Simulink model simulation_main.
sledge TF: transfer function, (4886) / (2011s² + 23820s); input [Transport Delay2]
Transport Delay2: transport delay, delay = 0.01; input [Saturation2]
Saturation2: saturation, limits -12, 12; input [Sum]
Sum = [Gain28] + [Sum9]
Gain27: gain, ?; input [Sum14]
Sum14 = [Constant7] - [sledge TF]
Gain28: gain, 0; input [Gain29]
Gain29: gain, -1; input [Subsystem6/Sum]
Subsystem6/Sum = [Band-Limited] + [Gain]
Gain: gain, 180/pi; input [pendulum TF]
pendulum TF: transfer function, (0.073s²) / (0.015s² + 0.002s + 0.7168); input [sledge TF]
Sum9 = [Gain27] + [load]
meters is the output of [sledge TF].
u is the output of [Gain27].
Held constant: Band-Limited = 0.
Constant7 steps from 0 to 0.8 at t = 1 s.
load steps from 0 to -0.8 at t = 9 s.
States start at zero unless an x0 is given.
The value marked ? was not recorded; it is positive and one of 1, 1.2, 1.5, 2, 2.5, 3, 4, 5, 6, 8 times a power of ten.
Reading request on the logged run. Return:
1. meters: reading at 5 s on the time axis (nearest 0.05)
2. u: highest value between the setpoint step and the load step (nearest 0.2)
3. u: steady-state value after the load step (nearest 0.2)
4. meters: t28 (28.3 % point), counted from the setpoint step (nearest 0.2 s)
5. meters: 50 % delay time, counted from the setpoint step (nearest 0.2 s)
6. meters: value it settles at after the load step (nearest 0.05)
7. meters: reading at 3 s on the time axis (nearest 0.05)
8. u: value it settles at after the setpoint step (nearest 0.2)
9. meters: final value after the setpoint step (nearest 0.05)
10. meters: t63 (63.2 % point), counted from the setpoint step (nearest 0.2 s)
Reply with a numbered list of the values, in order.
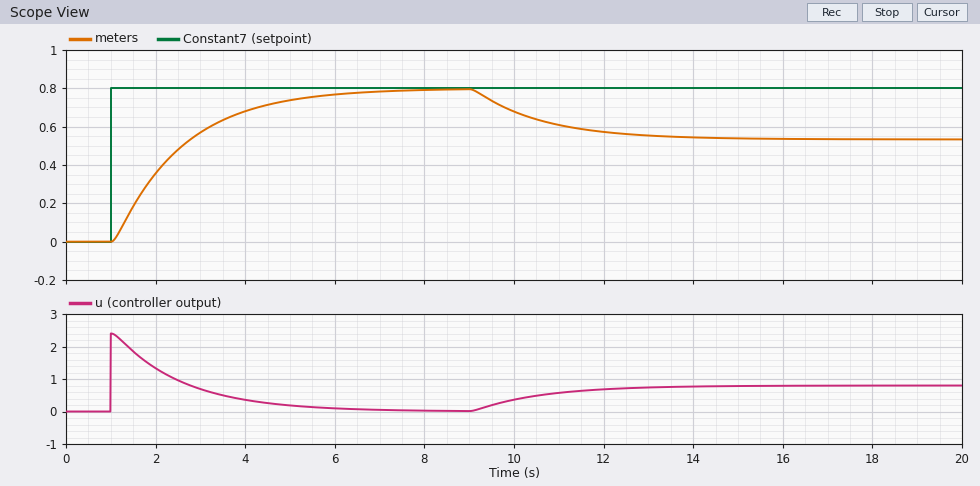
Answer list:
1. 0.75
2. 2.4
3. 0.8
4. 0.6 s
5. 1.2 s
6. 0.55
7. 0.55
8. 0.0
9. 0.80
10. 1.6 s
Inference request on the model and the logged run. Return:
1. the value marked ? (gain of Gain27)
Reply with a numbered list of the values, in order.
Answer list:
1. 3
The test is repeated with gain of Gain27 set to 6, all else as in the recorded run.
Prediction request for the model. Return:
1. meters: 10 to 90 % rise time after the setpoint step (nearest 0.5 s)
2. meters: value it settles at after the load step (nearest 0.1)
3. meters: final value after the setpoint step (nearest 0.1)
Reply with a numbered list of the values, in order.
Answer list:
1. 1.5 s
2. 0.7
3. 0.8
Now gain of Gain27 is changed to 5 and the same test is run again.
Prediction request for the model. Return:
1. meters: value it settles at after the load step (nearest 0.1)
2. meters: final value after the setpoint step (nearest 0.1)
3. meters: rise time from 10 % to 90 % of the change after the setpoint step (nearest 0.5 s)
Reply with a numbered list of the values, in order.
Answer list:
1. 0.6
2. 0.8
3. 2.0 s
